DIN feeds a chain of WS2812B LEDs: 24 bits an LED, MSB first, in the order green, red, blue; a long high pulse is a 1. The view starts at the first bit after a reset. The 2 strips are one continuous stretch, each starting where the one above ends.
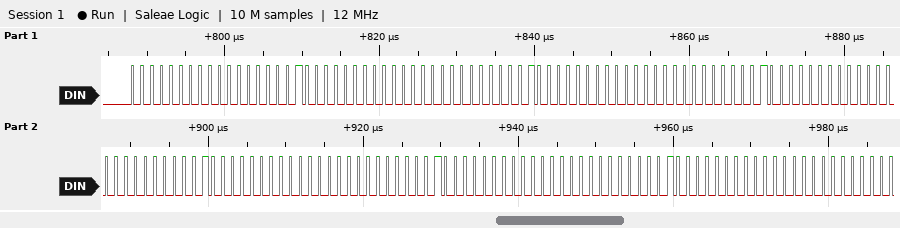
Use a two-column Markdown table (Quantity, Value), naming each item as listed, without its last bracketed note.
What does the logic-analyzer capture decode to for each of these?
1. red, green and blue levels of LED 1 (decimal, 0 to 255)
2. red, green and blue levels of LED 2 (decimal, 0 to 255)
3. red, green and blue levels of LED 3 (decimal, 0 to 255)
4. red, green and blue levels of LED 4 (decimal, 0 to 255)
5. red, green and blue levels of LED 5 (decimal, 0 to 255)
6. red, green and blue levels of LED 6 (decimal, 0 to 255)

| Quantity | Value |
|---|---|
| red, green and blue levels of LED 1 | 0, 0, 64 |
| red, green and blue levels of LED 2 | 0, 0, 64 |
| red, green and blue levels of LED 3 | 0, 0, 64 |
| red, green and blue levels of LED 4 | 0, 0, 64 |
| red, green and blue levels of LED 5 | 0, 0, 64 |
| red, green and blue levels of LED 6 | 0, 0, 64 |
